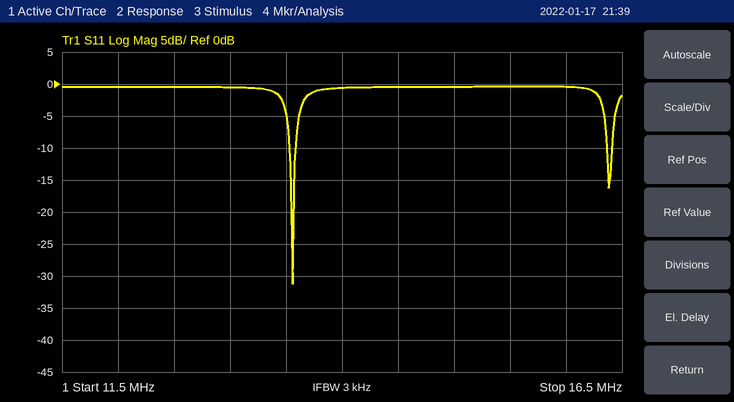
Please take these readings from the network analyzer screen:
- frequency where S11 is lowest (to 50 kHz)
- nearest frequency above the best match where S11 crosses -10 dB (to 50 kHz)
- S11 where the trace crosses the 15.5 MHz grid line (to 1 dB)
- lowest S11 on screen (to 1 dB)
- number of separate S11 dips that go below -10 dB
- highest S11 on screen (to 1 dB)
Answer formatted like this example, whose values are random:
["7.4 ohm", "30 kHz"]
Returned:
["13.55 MHz", "13.60 MHz", "0 dB", "-31 dB", "2", "0 dB"]
